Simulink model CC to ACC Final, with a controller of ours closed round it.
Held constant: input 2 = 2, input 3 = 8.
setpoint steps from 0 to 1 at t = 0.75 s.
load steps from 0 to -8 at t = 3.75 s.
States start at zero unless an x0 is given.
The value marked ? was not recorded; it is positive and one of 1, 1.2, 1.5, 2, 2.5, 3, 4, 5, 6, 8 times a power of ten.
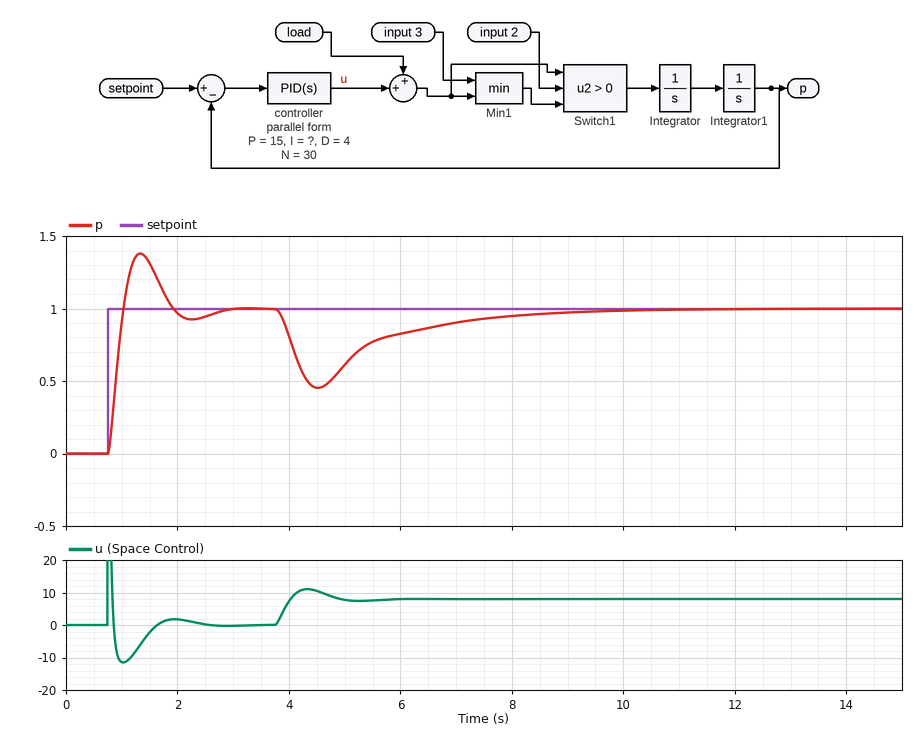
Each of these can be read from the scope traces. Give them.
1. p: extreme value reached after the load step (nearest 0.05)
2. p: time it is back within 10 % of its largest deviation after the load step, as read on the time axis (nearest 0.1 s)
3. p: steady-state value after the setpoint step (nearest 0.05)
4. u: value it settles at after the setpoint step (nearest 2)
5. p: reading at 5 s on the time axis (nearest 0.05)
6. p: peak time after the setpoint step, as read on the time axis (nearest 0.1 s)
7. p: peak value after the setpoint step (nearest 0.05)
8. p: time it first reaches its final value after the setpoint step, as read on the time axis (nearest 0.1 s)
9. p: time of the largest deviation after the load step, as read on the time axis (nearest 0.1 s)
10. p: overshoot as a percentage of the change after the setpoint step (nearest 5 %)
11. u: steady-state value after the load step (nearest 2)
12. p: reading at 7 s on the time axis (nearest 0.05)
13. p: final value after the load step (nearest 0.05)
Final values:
0.45
7.9 s
1.00
0
0.60
1.3 s
1.40
1.0 s
4.5 s
40 %
8
0.90
1.00
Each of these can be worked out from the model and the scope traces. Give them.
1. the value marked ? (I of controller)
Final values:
8
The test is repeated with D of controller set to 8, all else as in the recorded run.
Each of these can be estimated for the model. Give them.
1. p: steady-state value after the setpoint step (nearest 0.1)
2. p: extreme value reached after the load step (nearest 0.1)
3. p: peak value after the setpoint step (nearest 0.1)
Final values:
1.0
0.6
1.2
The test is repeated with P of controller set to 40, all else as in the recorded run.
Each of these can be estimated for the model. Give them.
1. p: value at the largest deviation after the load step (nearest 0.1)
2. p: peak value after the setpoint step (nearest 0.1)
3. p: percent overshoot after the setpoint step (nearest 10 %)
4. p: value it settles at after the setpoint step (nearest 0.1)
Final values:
0.7
1.5
50 %
1.0
